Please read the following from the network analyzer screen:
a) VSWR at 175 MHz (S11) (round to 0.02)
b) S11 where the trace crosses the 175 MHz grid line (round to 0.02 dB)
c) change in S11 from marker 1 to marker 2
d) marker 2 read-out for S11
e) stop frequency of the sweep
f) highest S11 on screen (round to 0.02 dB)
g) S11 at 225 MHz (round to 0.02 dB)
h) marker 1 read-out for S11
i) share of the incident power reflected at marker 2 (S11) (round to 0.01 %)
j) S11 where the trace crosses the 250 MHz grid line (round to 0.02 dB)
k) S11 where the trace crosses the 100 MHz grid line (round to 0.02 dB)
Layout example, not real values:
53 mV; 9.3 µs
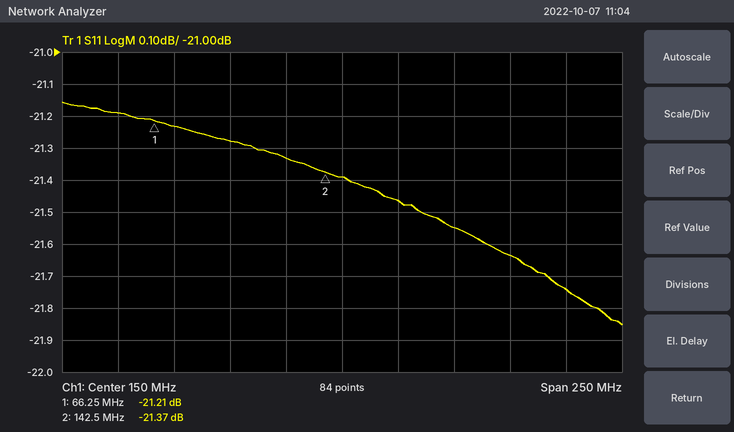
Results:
1.18; -21.46 dB; -0.16 dB; -21.37 dB; 275 MHz; -21.16 dB; -21.64 dB; -21.21 dB; 0.73 %; -21.74 dB; -21.28 dB
